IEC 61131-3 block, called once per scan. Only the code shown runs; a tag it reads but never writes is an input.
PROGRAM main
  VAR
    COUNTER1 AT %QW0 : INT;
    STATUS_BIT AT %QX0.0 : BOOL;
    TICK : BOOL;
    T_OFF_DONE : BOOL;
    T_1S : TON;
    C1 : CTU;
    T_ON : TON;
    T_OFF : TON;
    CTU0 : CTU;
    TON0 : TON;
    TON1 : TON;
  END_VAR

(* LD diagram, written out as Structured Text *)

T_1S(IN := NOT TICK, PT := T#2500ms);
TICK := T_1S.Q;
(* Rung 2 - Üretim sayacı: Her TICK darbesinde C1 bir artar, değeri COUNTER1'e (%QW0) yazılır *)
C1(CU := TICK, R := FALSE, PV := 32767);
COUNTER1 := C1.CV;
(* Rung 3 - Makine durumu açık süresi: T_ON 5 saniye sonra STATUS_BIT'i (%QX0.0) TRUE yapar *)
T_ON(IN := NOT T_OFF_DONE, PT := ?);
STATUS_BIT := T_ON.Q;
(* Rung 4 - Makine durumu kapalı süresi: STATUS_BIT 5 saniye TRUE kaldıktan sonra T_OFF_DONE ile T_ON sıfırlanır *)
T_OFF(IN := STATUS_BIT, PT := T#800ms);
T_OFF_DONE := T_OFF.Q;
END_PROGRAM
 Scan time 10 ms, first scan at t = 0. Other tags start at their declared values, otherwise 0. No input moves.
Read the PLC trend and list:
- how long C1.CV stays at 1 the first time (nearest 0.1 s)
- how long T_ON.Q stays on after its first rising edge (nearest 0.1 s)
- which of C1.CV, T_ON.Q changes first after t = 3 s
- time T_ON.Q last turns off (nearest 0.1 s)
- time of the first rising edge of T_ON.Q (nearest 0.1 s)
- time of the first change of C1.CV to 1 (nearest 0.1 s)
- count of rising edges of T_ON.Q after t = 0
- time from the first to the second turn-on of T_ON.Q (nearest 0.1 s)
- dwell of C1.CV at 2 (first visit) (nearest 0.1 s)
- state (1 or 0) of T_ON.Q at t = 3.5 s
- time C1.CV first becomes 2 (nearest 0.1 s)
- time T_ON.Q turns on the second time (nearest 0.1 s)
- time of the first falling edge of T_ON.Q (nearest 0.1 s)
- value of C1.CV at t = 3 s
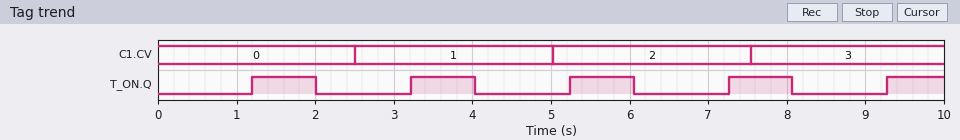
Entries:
2.5 s
0.8 s
T_ON.Q
8.1 s
1.2 s
2.5 s
5
2.0 s
2.5 s
1
5.0 s
3.2 s
2.0 s
1
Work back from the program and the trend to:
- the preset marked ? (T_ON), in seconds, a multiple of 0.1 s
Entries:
1.2 s
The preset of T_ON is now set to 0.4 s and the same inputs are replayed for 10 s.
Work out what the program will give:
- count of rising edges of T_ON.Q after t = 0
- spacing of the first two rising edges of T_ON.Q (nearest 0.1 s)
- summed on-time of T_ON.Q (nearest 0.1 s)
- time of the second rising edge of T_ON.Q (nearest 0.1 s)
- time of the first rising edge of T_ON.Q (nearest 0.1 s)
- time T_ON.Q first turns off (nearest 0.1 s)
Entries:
8
1.2 s
6.5 s
1.6 s
0.4 s
1.2 s
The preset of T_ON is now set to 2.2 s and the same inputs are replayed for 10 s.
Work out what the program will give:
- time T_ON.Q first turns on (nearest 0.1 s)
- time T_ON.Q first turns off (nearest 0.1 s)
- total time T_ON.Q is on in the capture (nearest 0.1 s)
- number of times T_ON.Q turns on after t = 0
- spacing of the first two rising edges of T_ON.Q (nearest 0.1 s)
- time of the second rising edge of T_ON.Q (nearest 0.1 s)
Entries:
2.2 s
3.0 s
2.4 s
3
3.0 s
5.2 s
